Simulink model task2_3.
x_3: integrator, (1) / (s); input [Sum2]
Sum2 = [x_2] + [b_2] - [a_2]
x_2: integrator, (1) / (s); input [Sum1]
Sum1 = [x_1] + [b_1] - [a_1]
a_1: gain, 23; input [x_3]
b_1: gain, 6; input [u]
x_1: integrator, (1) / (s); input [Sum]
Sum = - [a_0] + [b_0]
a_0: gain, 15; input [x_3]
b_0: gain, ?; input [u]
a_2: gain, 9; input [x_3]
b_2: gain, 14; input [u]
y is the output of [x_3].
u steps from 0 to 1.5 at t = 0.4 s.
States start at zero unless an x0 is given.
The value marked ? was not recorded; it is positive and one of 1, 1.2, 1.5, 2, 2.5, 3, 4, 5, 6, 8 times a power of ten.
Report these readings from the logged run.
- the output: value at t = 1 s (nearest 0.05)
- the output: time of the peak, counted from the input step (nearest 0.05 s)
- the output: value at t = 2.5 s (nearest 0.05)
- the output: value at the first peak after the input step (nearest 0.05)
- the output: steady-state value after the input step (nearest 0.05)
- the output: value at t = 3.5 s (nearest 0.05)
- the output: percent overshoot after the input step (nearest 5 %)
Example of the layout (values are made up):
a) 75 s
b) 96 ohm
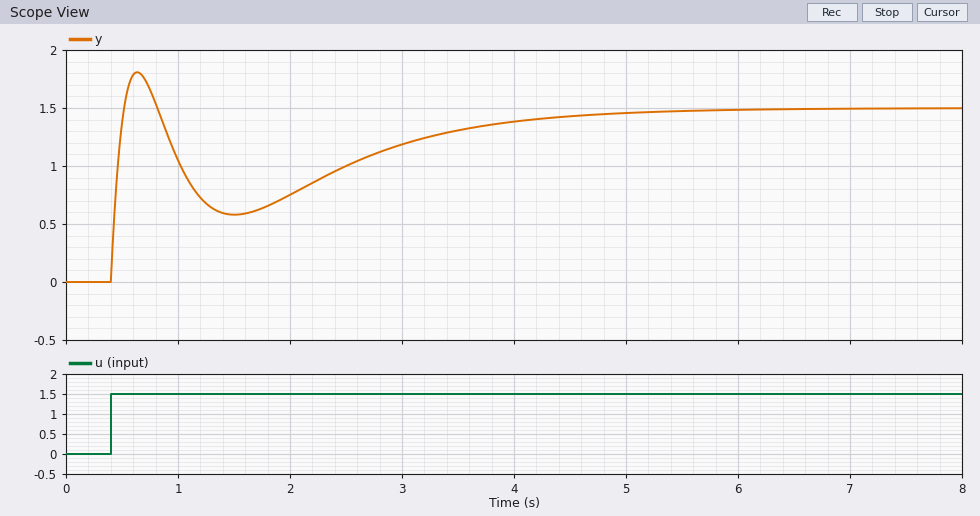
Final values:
a) 1.05
b) 0.25 s
c) 1.00
d) 1.80
e) 1.50
f) 1.30
g) 20 %
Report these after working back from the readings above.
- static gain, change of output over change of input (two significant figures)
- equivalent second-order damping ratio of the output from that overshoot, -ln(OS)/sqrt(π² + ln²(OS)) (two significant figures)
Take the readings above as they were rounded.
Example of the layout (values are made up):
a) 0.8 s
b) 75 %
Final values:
a) 1.0
b) 0.46
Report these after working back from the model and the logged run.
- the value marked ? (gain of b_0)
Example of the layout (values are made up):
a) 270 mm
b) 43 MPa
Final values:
a) 15
